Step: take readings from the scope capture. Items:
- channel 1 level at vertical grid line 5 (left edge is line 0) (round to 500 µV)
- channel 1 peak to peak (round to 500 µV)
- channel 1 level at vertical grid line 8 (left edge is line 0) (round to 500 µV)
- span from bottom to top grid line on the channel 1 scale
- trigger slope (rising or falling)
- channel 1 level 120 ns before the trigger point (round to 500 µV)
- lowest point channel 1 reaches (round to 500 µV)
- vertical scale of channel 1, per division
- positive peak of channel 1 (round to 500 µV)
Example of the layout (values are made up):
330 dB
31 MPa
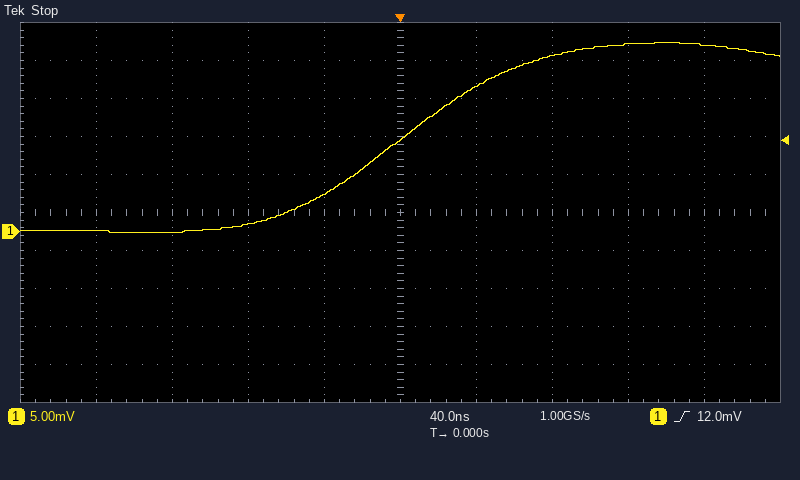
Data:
12.0 mV
25.0 mV
24.5 mV
50 mV
rising
0.0 mV
0.0 mV
5 mV
25.0 mV
